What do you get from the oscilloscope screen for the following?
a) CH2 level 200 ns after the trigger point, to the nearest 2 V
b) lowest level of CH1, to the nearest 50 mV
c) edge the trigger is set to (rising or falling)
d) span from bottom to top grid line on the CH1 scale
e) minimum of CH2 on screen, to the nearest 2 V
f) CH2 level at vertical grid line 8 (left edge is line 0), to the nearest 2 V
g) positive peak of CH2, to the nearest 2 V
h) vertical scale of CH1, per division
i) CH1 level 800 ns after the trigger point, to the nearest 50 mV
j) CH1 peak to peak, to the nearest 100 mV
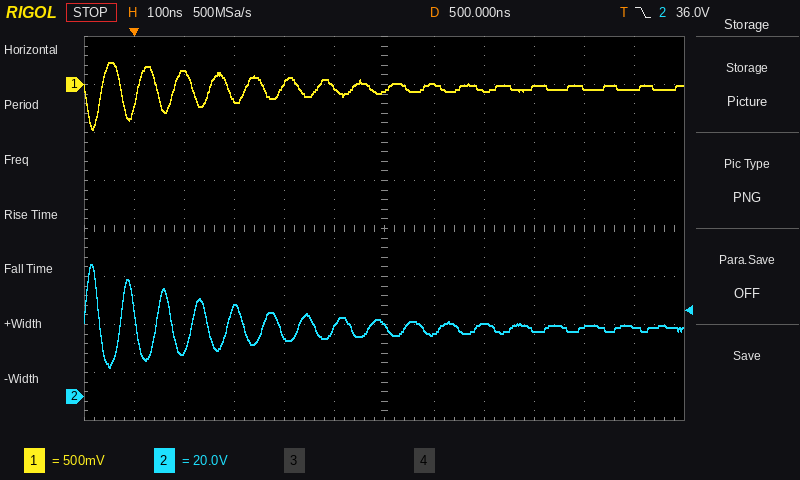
36 V
-450 mV
falling
4 V
12 V
30 V
56 V
500 mV
-50 mV
700 mV
